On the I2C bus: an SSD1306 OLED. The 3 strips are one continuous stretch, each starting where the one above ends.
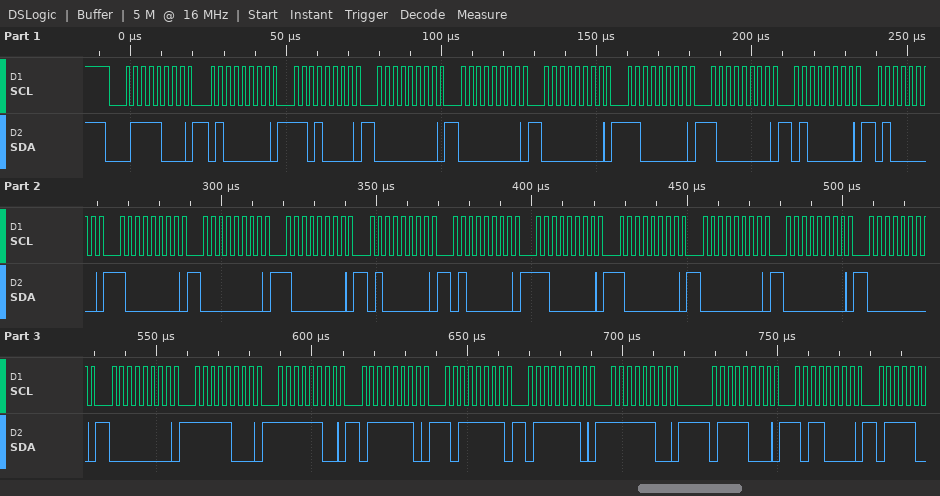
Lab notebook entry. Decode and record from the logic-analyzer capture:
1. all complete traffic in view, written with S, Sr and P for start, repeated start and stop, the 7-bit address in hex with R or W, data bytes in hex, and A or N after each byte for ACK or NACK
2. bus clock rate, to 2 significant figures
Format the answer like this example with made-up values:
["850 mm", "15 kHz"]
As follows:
["S 3CW A 40 A D0 A 00 A 00 A 00 A C0 A 80 A 40 A 40 A 80 A 00 A 80 A 40 A 40 A C0 A 80 A 00 A 00 A 00 A 00 A F8 A FC A 7E A BF A 7E A FC A 78 A B0 A", "400 kHz"]
